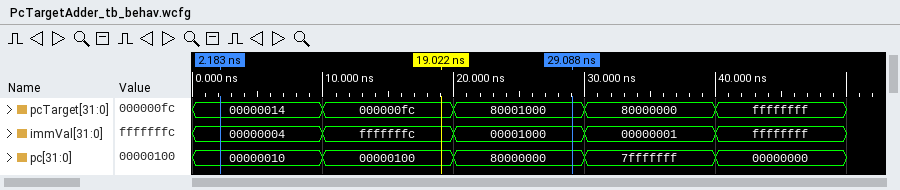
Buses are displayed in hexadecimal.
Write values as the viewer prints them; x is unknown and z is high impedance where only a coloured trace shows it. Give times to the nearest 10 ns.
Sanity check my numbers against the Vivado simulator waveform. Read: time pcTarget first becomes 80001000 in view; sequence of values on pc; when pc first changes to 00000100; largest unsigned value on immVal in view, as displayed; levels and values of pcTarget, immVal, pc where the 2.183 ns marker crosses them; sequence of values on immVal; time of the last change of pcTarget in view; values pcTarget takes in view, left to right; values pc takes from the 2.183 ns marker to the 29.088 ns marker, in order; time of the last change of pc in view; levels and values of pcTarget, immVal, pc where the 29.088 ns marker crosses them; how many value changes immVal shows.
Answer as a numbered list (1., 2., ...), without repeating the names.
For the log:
1. 20 ns
2. 00000010, 00000100, 80000000, 7fffffff, 00000000
3. 10 ns
4. ffffffff
5. pcTarget=00000014, immVal=00000004, pc=00000010
6. 00000004, fffffffc, 00001000, 00000001, ffffffff
7. 40 ns
8. 00000014, 000000fc, 80001000, 80000000, ffffffff
9. 00000010, 00000100, 80000000
10. 40 ns
11. pcTarget=80001000, immVal=00001000, pc=80000000
12. 4
